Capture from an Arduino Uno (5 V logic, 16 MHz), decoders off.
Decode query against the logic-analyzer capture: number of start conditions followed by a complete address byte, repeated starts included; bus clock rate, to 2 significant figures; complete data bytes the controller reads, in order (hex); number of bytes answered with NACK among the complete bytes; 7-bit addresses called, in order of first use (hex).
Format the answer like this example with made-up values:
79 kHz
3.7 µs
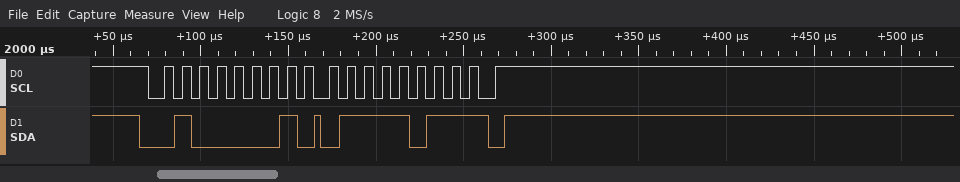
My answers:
1
100 kHz
7B
1
0x20
